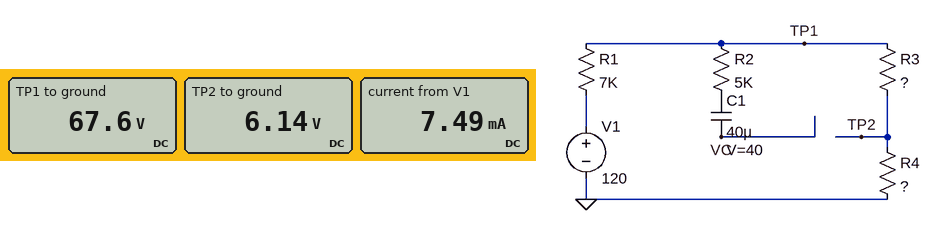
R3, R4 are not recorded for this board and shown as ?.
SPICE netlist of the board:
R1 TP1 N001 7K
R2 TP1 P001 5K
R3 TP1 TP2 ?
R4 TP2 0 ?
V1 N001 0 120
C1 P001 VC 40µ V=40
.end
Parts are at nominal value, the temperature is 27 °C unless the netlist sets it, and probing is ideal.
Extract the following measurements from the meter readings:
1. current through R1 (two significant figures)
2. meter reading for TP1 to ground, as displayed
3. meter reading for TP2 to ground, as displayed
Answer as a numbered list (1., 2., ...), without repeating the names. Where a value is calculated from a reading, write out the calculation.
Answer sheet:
1. (120 V - 67.6 V) / 7 kΩ = 7.5 mA
2. 67.6 V
3. 6.14 V
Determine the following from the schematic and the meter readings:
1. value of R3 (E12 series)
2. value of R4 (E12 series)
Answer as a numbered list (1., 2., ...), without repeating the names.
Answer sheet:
1. 8.2 kΩ
2. 820 Ω
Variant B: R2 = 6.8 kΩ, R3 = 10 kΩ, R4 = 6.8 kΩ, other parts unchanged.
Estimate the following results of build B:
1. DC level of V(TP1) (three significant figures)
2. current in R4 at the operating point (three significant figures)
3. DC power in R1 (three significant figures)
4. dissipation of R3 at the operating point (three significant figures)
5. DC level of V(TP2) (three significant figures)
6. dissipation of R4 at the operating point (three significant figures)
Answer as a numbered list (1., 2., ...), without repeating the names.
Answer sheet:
1. 84.7 V
2. 5.04 mA
3. 178 mW
4. 254 mW
5. 34.3 V
6. 173 mW
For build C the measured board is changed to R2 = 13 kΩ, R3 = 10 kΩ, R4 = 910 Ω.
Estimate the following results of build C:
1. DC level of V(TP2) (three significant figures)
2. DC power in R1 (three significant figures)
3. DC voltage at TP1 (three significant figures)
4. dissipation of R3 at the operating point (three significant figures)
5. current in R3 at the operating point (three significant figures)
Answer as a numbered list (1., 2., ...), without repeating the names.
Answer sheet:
1. 6.10 V
2. 314 mW
3. 73.1 V
4. 449 mW
5. 6.70 mA
